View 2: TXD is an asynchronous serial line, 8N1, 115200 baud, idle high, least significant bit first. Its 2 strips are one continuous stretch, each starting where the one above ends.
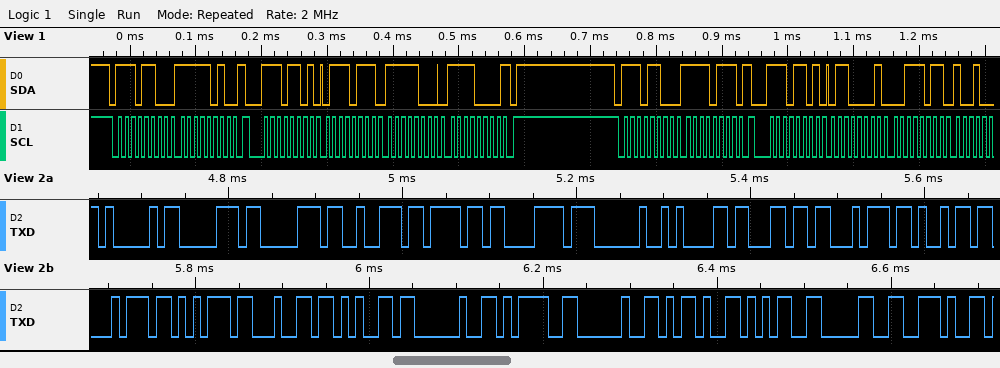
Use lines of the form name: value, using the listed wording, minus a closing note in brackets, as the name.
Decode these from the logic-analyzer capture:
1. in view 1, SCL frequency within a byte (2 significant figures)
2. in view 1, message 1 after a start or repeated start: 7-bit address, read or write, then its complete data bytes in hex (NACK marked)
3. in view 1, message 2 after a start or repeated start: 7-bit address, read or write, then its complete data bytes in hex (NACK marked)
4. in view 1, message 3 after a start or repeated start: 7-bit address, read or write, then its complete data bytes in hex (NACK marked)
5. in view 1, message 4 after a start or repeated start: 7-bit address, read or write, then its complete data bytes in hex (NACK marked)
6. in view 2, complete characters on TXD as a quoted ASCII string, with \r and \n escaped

in view 1, SCL frequency within a byte: 100 kHz
in view 1, message 1 after a start or repeated start: 7-bit address, read or write, then its complete data bytes in hex: 0x76 write: FA
in view 1, message 2 after a start or repeated start: 7-bit address, read or write, then its complete data bytes in hex: 0x76 read: 77 F8 F0 NACK
in view 1, message 3 after a start or repeated start: 7-bit address, read or write, then its complete data bytes in hex: 0x76 write: F7
in view 1, message 4 after a start or repeated start: 7-bit address, read or write, then its complete data bytes in hex: 0x76 read: 61 3B
in view 2, complete characters on TXD as a quoted ASCII string, with \r and \n escaped: "Approx altitude = -50."
